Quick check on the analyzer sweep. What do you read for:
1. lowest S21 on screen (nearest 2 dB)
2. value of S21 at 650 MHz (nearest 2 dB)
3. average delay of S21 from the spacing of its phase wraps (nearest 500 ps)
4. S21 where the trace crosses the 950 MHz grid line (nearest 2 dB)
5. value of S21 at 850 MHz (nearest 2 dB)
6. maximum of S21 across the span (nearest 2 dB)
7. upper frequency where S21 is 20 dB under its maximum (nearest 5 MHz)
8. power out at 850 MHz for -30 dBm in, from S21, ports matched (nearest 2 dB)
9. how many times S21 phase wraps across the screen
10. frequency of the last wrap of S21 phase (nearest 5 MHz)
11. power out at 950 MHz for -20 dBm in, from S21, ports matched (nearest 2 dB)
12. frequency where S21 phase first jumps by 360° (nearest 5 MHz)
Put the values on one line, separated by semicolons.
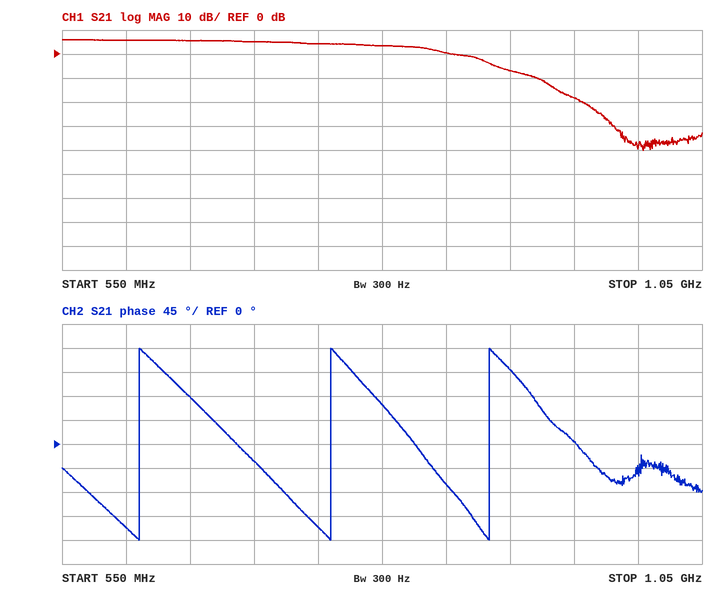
-40 dB; 6 dB; 7.5 ns; -18 dB; 0 dB; 6 dB; 935 MHz; -30 dBm; 3; 885 MHz; -38 dBm; 610 MHz
